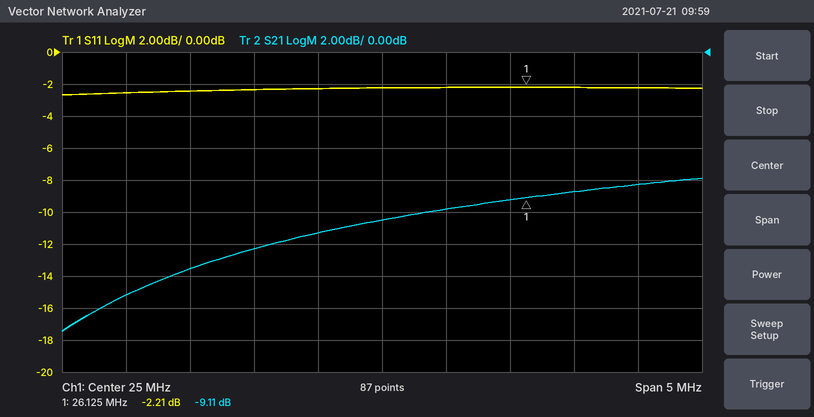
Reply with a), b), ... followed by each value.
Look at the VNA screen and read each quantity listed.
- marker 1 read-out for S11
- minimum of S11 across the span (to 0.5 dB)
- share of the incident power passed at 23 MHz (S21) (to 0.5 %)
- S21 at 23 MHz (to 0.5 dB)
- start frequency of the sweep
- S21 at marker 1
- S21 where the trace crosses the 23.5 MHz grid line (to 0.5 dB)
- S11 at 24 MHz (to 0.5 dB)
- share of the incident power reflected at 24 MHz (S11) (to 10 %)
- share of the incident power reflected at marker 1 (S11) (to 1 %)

a) -2.21 dB
b) -2.5 dB
c) 3.0 %
d) -15.0 dB
e) 22.5 MHz
f) -9.11 dB
g) -13.5 dB
h) -2.5 dB
i) 60 %
j) 60 %
